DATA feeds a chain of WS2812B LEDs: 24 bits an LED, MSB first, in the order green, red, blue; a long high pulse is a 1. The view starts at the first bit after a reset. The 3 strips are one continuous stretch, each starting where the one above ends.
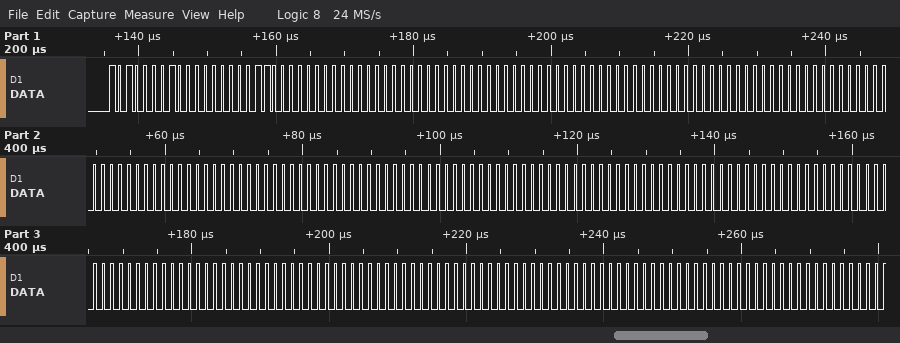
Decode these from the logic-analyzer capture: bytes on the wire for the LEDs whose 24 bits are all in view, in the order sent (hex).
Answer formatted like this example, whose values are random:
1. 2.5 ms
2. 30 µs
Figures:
1. A1 00 60 00 00 00 00 00 00 00 00 00 00 00 00 00 00 00 00 00 00 00 00 00 00 00 00 00 00 00 00 00 00
